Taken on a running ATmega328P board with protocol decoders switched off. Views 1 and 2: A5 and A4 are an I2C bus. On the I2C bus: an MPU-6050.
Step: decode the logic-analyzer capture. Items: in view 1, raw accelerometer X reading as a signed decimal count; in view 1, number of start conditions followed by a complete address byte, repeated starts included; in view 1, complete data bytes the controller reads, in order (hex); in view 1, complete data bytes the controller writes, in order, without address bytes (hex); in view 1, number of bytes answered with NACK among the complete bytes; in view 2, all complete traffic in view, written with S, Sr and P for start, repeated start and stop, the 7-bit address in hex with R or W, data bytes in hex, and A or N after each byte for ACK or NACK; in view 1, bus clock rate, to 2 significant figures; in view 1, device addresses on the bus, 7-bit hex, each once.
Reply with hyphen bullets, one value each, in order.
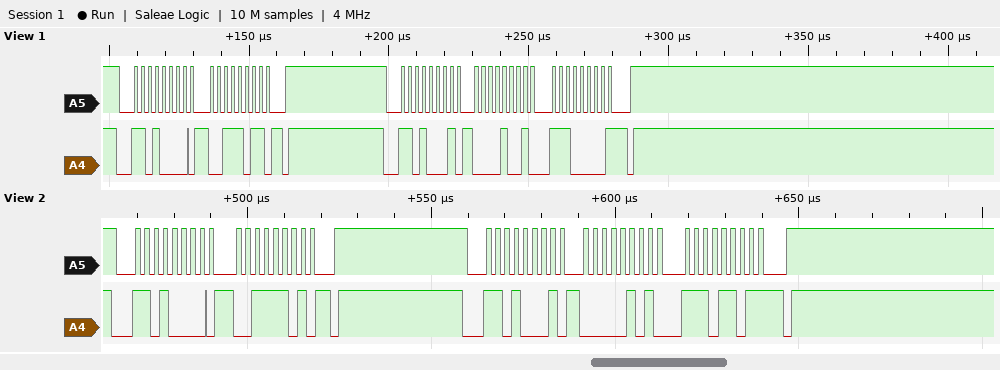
- 2528
- 2
- 09 E0
- 3B
- 1
- S 68W A 3D A P S 68R A 05 A ED N P
- 400 kHz
- 0x68
